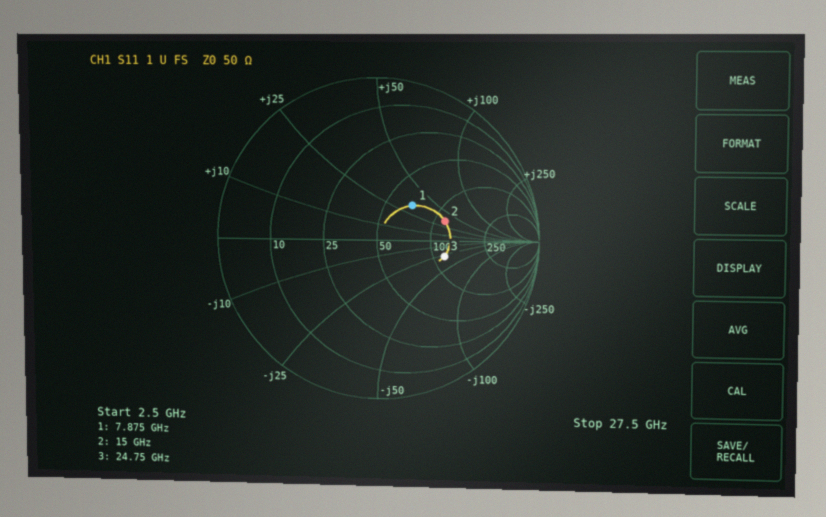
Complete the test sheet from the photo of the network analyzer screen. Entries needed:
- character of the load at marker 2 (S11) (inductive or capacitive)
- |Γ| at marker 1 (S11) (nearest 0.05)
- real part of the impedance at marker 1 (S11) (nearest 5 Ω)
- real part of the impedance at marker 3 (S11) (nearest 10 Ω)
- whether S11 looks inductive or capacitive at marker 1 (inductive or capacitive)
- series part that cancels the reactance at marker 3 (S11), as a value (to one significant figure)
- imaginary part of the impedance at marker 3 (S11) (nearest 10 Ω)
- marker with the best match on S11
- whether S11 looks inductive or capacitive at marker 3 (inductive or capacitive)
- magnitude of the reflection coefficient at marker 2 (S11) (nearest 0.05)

inductive
0.30
70 Ω
120 Ω
inductive
200 pH
-30 Ω
marker 1
capacitive
0.45
